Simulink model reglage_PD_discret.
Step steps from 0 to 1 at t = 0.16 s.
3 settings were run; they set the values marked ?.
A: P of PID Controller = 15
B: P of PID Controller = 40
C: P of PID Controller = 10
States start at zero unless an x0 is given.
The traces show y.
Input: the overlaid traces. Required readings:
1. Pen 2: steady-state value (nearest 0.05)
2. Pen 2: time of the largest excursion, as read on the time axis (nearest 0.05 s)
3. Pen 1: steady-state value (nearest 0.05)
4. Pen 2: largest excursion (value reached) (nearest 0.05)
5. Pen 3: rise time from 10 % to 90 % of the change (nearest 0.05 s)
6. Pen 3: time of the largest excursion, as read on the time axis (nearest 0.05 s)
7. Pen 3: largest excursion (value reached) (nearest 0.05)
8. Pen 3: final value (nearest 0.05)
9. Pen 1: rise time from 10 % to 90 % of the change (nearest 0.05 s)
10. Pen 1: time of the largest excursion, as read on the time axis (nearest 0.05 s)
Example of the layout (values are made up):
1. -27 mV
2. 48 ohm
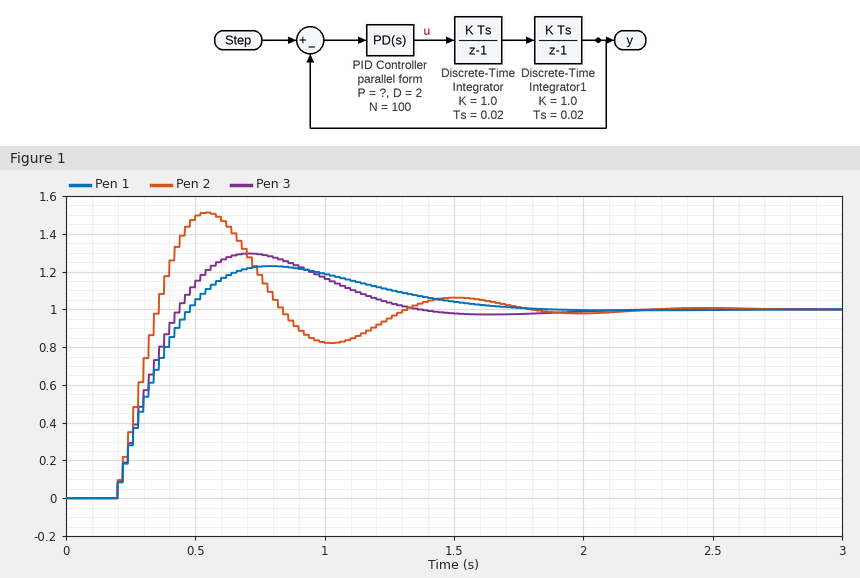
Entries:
1. 1.00
2. 0.55 s
3. 1.00
4. 1.50
5. 0.20 s
6. 0.70 s
7. 1.30
8. 1.00
9. 0.20 s
10. 0.80 s
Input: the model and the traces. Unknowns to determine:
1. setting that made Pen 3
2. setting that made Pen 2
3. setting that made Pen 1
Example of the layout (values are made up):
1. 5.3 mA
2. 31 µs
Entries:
1. A
2. B
3. C
